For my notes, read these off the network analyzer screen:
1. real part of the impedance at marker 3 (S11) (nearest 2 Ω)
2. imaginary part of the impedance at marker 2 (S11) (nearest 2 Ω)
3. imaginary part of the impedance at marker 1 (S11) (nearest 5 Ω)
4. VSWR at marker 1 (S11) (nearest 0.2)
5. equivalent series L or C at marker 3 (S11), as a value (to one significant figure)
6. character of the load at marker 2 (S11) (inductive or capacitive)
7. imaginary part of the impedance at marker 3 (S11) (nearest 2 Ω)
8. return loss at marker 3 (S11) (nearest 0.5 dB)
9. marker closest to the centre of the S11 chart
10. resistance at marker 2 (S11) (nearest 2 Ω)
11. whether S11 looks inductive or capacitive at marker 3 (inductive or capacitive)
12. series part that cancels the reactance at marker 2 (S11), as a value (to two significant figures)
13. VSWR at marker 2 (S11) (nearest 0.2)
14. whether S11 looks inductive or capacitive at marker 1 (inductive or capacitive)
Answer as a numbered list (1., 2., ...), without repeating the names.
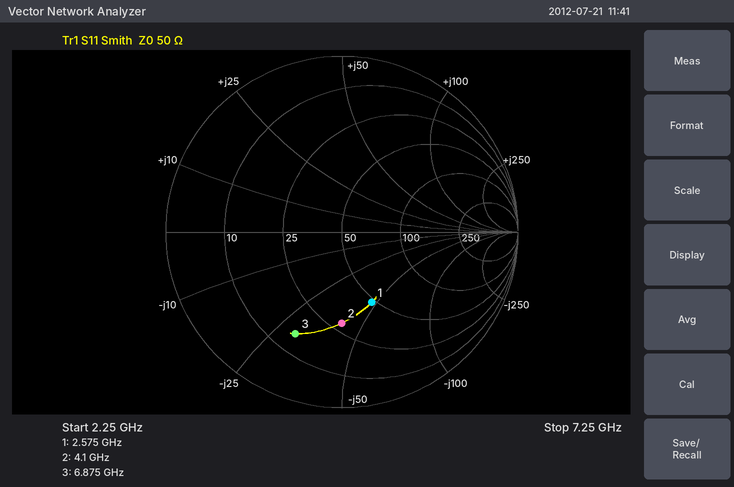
1. 16 Ω
2. -40 Ω
3. -45 Ω
4. 2.6
5. 800 fF
6. capacitive
7. -30 Ω
8. 4.0 dB
9. marker 1
10. 28 Ω
11. capacitive
12. 1.6 nH
13. 3.2
14. capacitive
